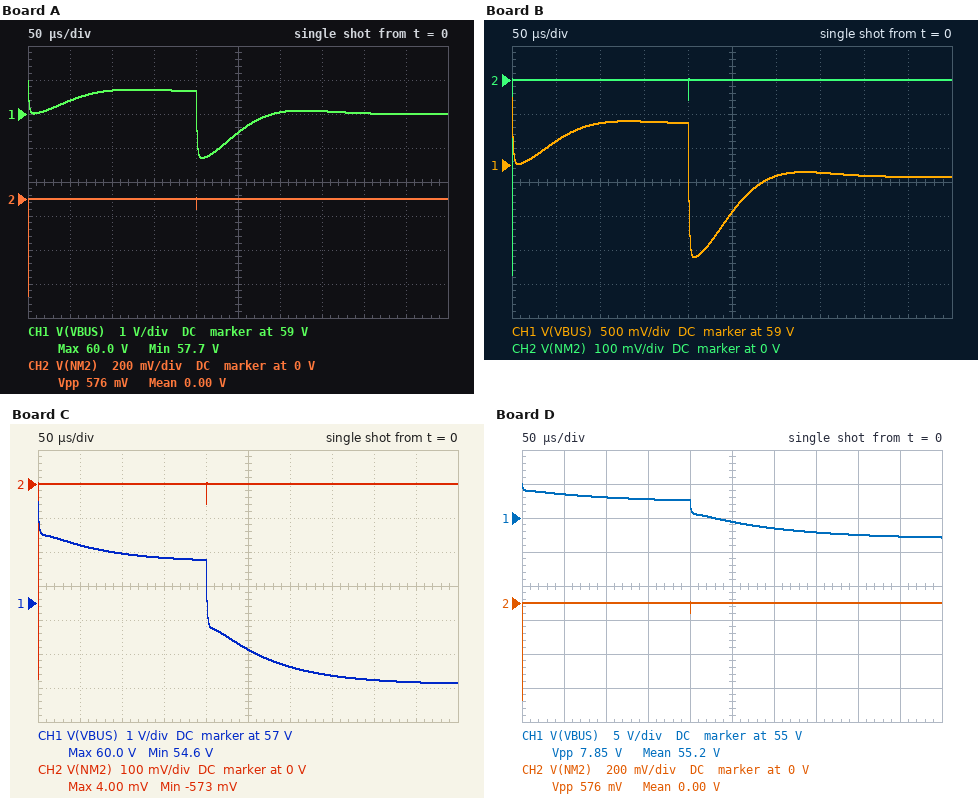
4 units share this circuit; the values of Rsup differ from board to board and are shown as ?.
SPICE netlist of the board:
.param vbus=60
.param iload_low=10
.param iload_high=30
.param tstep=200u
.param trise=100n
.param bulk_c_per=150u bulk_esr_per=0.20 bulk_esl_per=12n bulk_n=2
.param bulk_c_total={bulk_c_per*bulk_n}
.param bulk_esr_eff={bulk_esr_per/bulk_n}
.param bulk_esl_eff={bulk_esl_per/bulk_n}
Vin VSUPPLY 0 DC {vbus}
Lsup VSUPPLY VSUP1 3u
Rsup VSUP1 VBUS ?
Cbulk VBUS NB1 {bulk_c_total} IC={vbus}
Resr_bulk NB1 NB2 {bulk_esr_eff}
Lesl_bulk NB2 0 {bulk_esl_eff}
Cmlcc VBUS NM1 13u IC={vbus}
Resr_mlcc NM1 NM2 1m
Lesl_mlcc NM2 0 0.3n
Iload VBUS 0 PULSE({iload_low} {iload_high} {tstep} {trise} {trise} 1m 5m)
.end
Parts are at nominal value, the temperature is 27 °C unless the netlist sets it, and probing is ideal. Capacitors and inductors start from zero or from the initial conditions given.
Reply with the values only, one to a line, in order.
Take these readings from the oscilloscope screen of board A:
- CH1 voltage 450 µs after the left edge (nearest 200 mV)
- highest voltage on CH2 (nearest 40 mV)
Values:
59.0 V
0 V
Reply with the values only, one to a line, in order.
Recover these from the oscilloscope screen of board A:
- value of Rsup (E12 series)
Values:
0.033 Ω
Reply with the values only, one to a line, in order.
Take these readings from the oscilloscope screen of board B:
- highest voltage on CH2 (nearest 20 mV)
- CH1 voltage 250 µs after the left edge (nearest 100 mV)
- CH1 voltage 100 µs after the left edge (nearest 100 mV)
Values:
0 V
58.3 V
59.6 V
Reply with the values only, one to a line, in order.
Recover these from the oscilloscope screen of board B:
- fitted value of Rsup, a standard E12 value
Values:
0.039 Ω
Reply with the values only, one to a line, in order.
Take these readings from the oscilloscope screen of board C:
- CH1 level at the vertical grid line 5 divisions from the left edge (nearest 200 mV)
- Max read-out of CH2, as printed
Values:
55.6 V
4.00 mV
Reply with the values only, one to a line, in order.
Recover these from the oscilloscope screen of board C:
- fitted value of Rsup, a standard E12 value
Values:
0.18 Ω
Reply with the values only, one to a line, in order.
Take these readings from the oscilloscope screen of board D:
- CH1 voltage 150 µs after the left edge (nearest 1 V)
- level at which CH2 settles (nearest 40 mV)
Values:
58 V
0 V
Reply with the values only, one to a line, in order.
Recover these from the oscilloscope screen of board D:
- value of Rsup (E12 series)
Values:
0.27 Ω
